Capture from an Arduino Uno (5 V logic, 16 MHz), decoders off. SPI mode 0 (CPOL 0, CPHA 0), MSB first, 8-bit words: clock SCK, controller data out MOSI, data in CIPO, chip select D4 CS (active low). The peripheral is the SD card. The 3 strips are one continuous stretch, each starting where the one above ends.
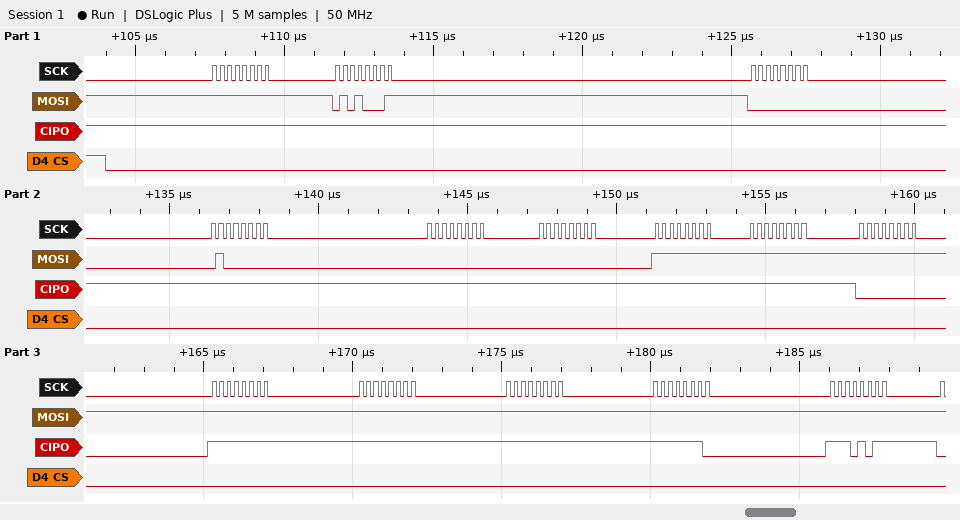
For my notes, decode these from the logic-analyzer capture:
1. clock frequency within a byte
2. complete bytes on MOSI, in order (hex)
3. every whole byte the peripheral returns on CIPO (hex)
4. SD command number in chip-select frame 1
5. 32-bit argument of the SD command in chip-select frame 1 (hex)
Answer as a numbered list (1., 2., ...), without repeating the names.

1. 4 MHz
2. 0xFF 0x51 0x00 0x40 0x00 0x00 0xFF 0xFF 0xFF 0xFF 0xFF 0xFF 0xFF 0xFF
3. 0xFF 0xFF 0xFF 0xFF 0xFF 0xFF 0xFF 0xFF 0x00 0xFF 0xFF 0xFF 0xFE 0xEB
4. CMD17
5. 0x00400000
